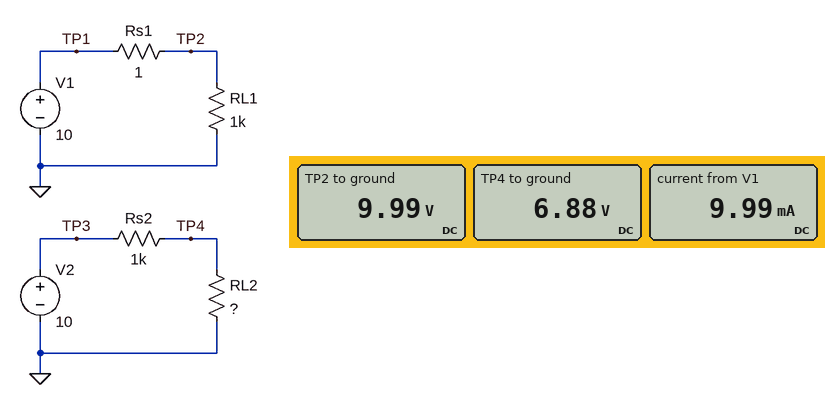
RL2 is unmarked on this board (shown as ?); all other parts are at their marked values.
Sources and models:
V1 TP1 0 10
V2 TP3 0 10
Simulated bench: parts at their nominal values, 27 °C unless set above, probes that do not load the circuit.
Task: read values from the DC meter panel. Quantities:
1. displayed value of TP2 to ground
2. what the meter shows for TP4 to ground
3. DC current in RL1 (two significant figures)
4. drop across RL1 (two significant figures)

9.99 V
6.88 V
10 mA
10 V
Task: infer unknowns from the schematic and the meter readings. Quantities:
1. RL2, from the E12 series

2.2 kΩ
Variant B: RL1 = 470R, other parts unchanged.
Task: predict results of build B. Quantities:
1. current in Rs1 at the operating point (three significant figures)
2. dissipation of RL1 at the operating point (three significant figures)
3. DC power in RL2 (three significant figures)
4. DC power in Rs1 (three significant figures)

21.2 mA
212 mW
21.5 mW
451 µW
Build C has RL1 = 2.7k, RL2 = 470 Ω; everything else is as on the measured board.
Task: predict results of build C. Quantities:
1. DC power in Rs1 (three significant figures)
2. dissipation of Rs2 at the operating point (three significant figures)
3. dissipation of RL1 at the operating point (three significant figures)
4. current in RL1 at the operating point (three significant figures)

13.7 µW
46.3 mW
37.0 mW
3.70 mA
